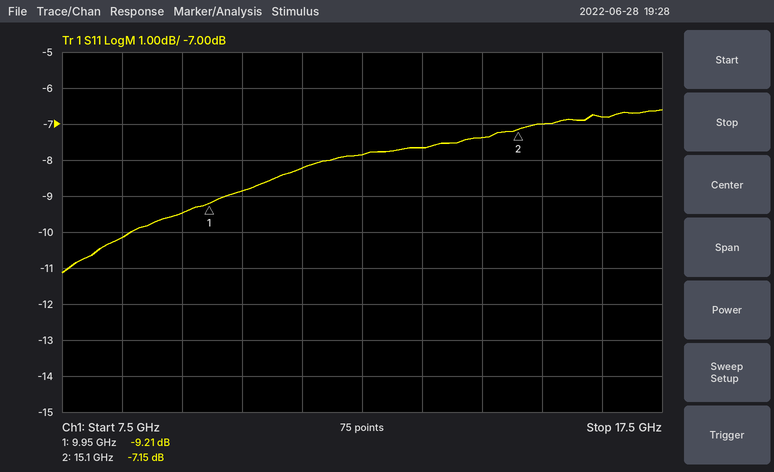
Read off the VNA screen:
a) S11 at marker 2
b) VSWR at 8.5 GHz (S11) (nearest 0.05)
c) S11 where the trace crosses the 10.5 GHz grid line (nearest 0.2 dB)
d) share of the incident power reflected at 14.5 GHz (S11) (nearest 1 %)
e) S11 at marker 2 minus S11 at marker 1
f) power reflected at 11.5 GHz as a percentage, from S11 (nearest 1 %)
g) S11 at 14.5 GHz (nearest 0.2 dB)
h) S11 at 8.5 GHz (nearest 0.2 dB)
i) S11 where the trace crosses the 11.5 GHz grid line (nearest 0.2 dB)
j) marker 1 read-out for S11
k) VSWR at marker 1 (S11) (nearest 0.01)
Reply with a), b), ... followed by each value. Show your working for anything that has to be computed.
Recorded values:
a) -7.15 dB
b) |Γ| = 10^(-10.2/20) = 0.3090; VSWR = (1 + 0.3090)/(1 − 0.3090) ≈ 1.89, so 1.90 to the nearest 0.05
c) -8.8 dB
d) 10^(-7.4/10) ≈ 18 %
e) -7.15 − (-9.21) = 2.06 dB
f) 10^(-8.2/10) ≈ 15 %
g) -7.4 dB
h) -10.2 dB
i) -8.2 dB
j) -9.21 dB
k) (1 + 0.3463)/(1 − 0.3463) ≈ 2.06
